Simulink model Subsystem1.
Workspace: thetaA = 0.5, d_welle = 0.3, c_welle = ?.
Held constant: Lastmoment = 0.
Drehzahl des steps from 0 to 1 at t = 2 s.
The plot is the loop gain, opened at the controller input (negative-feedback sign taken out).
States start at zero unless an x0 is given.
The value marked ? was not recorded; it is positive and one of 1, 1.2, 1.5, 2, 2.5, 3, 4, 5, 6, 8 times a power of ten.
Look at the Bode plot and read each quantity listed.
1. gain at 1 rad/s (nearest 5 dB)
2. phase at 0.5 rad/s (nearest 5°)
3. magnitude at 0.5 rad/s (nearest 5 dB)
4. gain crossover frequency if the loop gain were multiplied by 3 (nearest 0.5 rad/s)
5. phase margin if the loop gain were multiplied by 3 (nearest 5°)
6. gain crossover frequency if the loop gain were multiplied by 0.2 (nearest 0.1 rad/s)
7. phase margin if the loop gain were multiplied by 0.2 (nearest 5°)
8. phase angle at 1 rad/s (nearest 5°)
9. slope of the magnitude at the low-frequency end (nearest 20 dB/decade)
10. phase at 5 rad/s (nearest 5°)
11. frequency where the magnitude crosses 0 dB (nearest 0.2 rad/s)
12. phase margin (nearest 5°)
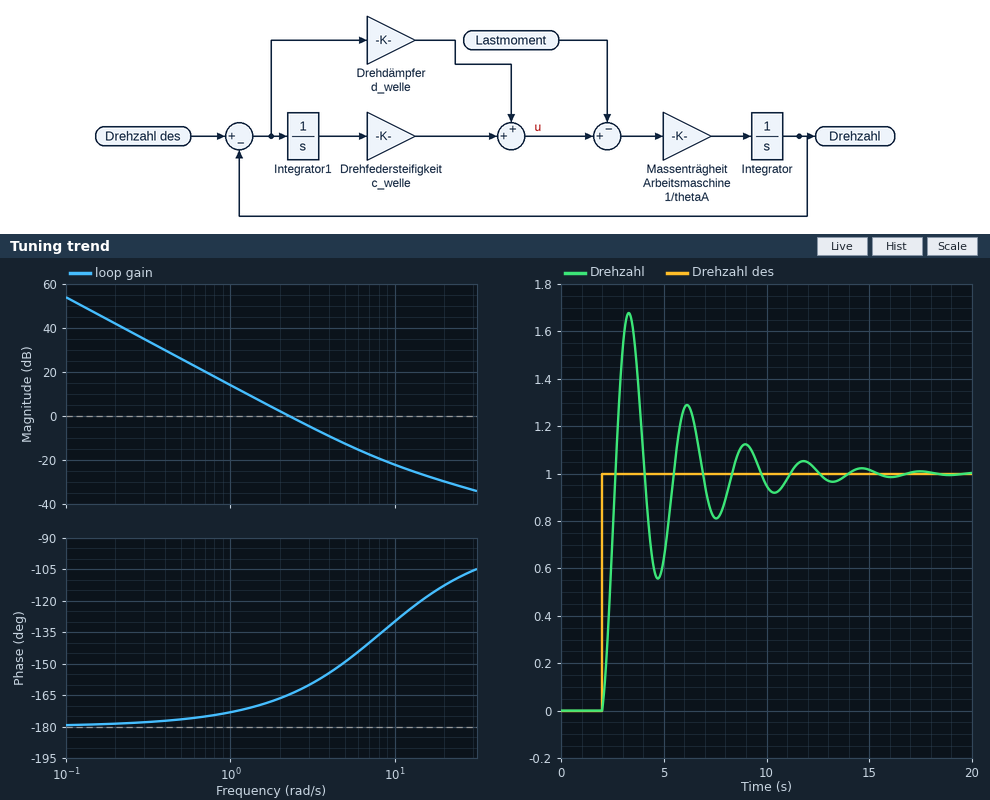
15 dB
-175°
25 dB
4.0 rad/s
25°
1.0 rad/s
5°
-175°
-40 dB/decade
-150°
2.2 rad/s
15°
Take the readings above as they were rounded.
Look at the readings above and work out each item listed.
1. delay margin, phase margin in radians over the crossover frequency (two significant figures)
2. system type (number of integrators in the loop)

0.12 s
2
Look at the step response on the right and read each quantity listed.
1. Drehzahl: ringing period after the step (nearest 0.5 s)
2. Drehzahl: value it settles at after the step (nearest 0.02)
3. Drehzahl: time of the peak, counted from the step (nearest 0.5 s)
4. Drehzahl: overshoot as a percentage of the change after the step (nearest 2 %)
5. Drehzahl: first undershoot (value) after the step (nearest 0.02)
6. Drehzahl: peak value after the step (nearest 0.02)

3.0 s
1.00
1.5 s
68 %
0.56
1.68
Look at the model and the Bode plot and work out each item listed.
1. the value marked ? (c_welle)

2.5
